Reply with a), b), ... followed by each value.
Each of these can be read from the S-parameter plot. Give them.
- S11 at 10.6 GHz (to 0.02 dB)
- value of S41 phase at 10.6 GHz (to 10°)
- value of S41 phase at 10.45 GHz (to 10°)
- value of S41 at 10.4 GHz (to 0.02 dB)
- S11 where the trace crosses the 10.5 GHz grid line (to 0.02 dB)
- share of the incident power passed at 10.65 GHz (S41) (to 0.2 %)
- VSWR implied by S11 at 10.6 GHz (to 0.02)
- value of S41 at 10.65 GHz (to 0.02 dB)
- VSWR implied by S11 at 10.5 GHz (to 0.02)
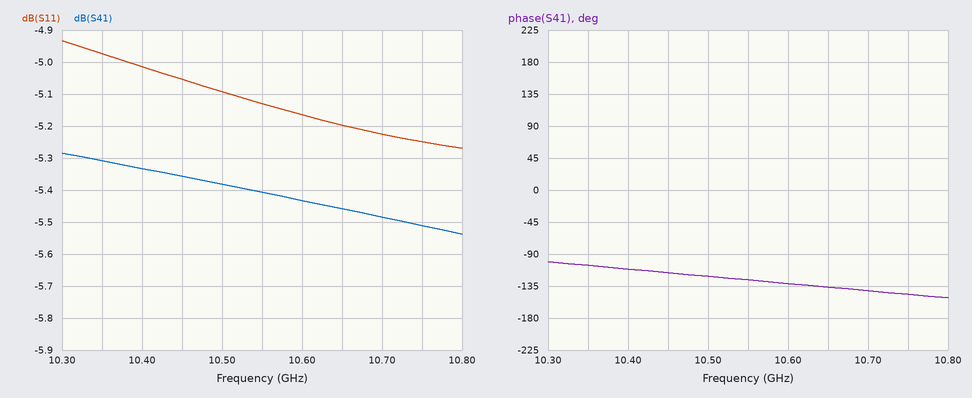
a) -5.16 dB
b) -130°
c) -120°
d) -5.34 dB
e) -5.10 dB
f) 28.4 %
g) 3.46
h) -5.46 dB
i) 3.50
